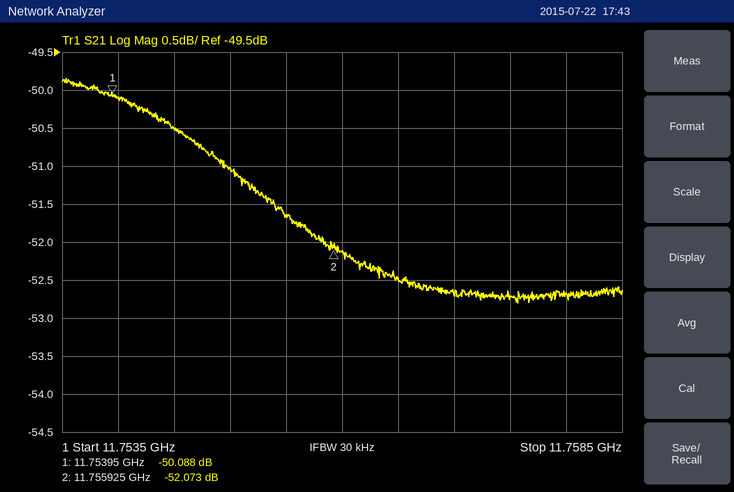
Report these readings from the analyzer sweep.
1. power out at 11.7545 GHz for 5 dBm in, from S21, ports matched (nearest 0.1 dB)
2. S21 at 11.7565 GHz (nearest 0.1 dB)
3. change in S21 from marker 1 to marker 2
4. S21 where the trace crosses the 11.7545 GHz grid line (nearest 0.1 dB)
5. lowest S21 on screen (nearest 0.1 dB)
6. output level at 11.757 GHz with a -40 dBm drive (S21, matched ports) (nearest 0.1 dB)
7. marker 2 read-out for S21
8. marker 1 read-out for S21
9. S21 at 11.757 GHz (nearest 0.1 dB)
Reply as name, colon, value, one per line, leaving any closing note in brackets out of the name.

power out at 11.7545 GHz for 5 dBm in, from S21, ports matched: -45.5 dBm
S21 at 11.7565 GHz: -52.5 dB
change in S21 from marker 1 to marker 2: -1.985 dB
S21 where the trace crosses the 11.7545 GHz grid line: -50.5 dB
lowest S21 on screen: -52.8 dB
output level at 11.757 GHz with a -40 dBm drive (S21, matched ports): -92.7 dBm
marker 2 read-out for S21: -52.073 dB
marker 1 read-out for S21: -50.088 dB
S21 at 11.757 GHz: -52.7 dB
